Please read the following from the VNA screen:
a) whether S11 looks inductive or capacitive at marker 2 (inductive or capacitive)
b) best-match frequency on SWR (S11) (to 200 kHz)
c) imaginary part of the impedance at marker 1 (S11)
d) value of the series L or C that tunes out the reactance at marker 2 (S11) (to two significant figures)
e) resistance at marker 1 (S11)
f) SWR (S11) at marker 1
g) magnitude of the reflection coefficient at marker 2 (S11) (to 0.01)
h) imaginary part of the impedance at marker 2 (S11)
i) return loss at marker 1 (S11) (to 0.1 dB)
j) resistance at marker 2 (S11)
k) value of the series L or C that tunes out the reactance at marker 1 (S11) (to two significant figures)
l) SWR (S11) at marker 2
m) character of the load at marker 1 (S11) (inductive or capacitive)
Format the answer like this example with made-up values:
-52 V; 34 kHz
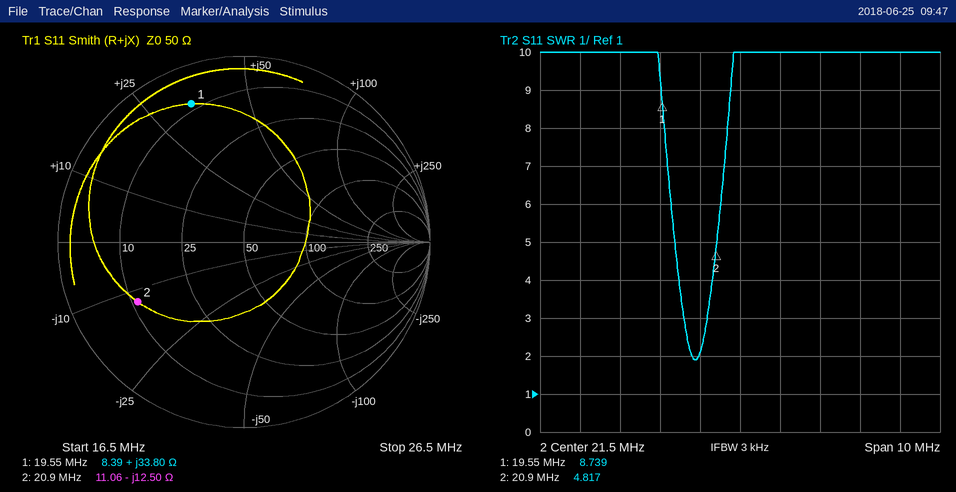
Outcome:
capacitive; 20.4 MHz; +33.80 Ω; 95 nH; 8.39 Ω; 8.739; 0.66; -12.50 Ω; 2.0 dB; 11.06 Ω; 240 pF; 4.817; inductive
